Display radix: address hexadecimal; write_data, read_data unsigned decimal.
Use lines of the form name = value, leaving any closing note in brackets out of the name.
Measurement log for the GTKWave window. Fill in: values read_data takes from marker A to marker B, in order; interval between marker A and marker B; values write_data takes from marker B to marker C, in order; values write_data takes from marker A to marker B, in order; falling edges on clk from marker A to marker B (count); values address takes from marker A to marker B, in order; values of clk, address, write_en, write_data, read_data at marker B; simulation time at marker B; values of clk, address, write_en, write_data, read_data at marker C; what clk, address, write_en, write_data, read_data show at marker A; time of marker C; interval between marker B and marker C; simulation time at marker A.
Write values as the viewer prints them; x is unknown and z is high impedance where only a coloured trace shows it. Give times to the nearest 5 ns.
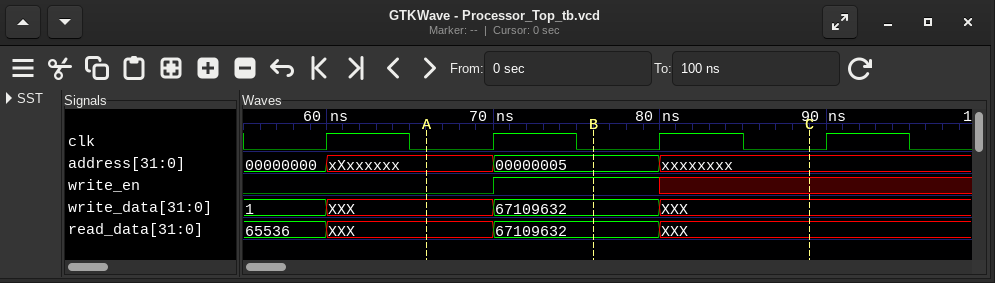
values read_data takes from marker A to marker B, in order = XXX, 67109632
interval between marker A and marker B = 10 ns
values write_data takes from marker B to marker C, in order = 67109632, XXX
values write_data takes from marker A to marker B, in order = XXX, 67109632
falling edges on clk from marker A to marker B = 1
values address takes from marker A to marker B, in order = xXxxxxxx, 00000005
values of clk, address, write_en, write_data, read_data at marker B = clk=0, address=00000005, write_en=1, write_data=67109632, read_data=67109632
simulation time at marker B = 75 ns
values of clk, address, write_en, write_data, read_data at marker C = clk=0, address=xxxxxxxx, write_en=x, write_data=XXX, read_data=XXX
what clk, address, write_en, write_data, read_data show at marker A = clk=0, address=xXxxxxxx, write_en=0, write_data=XXX, read_data=XXX
time of marker C = 90 ns
interval between marker B and marker C = 15 ns
simulation time at marker A = 65 ns
